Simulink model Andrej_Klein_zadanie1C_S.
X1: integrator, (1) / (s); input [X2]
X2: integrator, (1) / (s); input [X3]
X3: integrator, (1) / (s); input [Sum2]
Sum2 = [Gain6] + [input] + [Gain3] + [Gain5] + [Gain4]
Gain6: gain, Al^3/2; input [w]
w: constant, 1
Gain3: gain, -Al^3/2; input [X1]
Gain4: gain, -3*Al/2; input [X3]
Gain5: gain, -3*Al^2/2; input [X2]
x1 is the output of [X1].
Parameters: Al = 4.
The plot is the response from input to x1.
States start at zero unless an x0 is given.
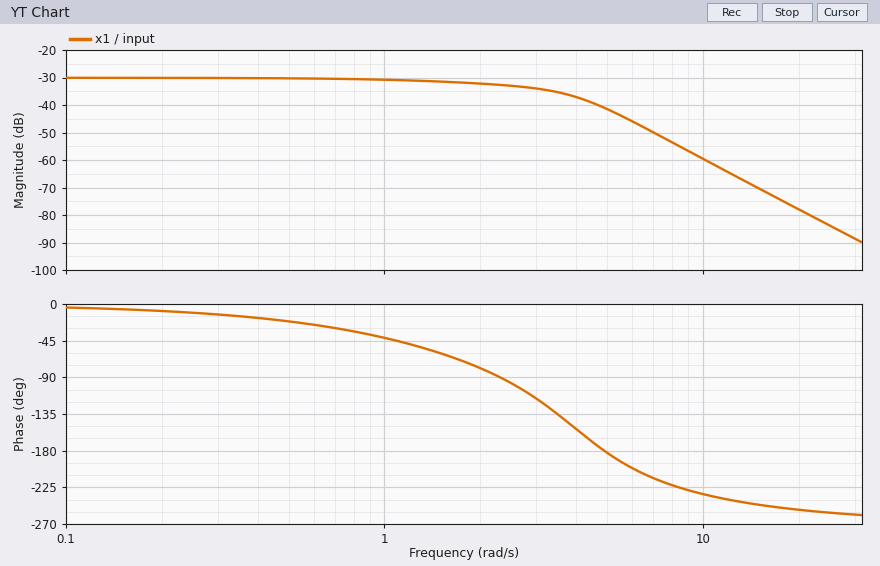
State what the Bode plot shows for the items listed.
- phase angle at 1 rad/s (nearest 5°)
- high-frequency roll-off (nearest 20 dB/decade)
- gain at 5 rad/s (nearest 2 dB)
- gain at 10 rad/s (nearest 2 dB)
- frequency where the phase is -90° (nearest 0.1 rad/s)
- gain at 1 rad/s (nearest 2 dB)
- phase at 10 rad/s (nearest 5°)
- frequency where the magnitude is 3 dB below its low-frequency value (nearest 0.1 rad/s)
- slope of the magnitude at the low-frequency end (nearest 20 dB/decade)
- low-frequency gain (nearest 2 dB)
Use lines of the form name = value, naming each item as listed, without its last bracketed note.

phase angle at 1 rad/s = -40°
high-frequency roll-off = -60 dB/decade
gain at 5 rad/s = -42 dB
gain at 10 rad/s = -60 dB
frequency where the phase is -90° = 2.3 rad/s
gain at 1 rad/s = -30 dB
phase at 10 rad/s = -235°
frequency where the magnitude is 3 dB below its low-frequency value = 2.6 rad/s
slope of the magnitude at the low-frequency end = 0 dB/decade
low-frequency gain = -30 dB
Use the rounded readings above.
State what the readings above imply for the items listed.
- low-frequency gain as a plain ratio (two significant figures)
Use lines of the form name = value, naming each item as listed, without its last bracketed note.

low-frequency gain as a plain ratio = 0.032
